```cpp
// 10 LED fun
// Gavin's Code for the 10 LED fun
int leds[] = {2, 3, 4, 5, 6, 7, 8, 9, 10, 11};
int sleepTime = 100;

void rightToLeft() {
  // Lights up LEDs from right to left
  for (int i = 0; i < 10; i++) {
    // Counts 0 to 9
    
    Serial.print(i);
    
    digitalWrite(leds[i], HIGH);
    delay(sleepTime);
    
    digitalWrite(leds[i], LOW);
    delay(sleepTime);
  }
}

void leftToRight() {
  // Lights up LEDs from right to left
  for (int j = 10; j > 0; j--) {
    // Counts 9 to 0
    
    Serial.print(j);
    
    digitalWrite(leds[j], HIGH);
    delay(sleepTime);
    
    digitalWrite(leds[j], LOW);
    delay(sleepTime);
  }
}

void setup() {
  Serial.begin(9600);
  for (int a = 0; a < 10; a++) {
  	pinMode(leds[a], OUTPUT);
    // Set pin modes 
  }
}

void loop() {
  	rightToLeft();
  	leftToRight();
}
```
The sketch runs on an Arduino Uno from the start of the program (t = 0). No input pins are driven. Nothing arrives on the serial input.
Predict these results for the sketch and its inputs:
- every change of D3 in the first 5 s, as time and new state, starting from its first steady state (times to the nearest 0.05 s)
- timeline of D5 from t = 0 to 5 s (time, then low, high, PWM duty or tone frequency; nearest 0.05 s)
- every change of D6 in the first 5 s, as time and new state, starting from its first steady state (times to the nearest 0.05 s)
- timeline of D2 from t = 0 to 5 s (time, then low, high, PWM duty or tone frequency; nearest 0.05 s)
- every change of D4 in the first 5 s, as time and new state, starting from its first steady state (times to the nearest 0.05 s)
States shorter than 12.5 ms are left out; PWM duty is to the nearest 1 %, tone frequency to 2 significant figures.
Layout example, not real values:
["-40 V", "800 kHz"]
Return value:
["0 s low; 0.2 s high; 0.3 s low; 3.8 s high; 3.9 s low; 4.2 s high; 4.3 s low", "0 s low; 0.6 s high; 0.7 s low; 3.4 s high; 3.5 s low; 4.6 s high; 4.7 s low", "0 s low; 0.8 s high; 0.9 s low; 3.2 s high; 3.3 s low; 4.8 s high; 4.9 s low", "0 s high; 0.1 s low; 4 s high; 4.1 s low", "0 s low; 0.4 s high; 0.5 s low; 3.6 s high; 3.7 s low; 4.4 s high; 4.5 s low"]
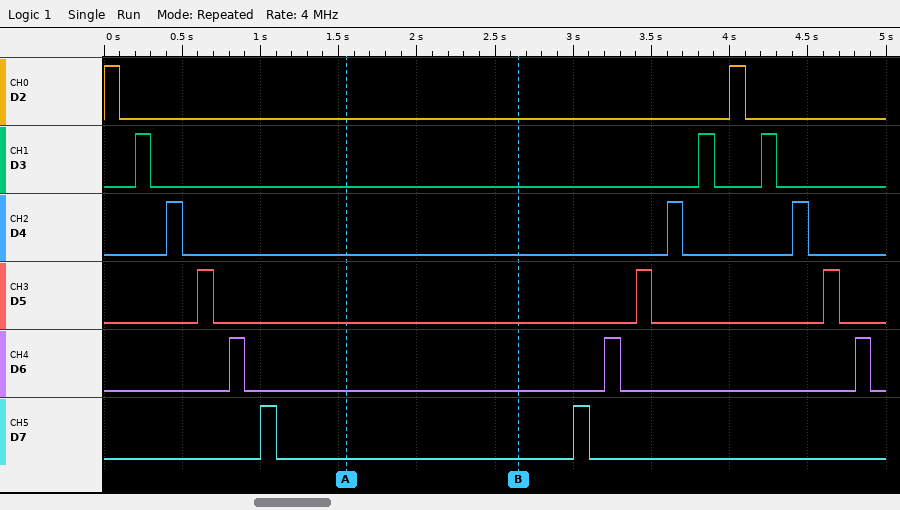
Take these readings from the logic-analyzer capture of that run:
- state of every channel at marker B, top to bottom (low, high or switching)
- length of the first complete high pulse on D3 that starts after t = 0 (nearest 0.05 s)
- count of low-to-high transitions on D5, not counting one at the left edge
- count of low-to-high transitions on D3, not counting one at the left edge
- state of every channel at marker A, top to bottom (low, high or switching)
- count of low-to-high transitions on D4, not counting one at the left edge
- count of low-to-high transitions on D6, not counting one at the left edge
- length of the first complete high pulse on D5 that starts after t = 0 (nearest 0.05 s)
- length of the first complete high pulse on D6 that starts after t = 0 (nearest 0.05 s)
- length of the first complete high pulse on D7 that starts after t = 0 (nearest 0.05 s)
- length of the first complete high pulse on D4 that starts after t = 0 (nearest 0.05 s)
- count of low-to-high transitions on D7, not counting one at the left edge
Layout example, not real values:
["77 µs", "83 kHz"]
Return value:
["D2 low, D3 low, D4 low, D5 low, D6 low, D7 low", "0.10 s", "3", "3", "D2 low, D3 low, D4 low, D5 low, D6 low, D7 low", "3", "3", "0.10 s", "0.10 s", "0.10 s", "0.10 s", "2"]
